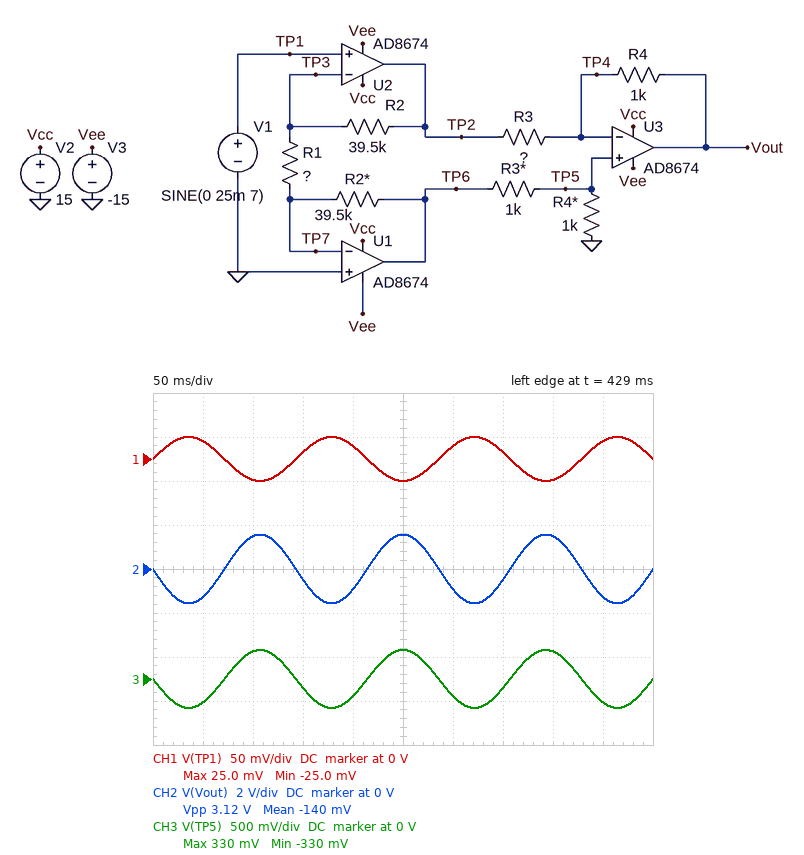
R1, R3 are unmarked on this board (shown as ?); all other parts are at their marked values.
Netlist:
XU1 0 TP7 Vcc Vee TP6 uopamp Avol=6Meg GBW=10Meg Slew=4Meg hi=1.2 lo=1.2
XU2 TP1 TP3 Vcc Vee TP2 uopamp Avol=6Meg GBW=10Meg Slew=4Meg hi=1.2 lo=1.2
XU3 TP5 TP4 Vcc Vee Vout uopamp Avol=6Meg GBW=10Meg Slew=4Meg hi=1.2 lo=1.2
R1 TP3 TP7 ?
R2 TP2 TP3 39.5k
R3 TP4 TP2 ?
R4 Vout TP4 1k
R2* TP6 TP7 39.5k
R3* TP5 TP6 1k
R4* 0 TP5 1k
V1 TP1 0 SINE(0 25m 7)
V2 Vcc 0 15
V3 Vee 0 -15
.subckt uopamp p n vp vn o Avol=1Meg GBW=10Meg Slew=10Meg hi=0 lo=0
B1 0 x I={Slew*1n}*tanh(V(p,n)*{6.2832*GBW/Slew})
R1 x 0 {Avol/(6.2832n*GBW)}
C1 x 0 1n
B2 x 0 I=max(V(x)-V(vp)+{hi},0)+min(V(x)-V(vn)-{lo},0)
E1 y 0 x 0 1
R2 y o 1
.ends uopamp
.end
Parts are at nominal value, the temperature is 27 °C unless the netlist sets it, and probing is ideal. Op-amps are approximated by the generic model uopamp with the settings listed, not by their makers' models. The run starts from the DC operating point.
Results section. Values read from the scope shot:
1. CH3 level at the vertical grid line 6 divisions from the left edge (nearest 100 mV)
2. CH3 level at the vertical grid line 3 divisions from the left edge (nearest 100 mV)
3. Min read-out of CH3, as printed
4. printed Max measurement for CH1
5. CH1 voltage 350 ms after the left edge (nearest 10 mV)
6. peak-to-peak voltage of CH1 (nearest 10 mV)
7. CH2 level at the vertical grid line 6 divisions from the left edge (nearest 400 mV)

-200 mV
-100 mV
-330 mV
25.0 mV
10 mV
50 mV
-800 mV
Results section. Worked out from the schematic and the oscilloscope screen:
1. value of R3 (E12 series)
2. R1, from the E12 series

820 Ω
1.5 kΩ
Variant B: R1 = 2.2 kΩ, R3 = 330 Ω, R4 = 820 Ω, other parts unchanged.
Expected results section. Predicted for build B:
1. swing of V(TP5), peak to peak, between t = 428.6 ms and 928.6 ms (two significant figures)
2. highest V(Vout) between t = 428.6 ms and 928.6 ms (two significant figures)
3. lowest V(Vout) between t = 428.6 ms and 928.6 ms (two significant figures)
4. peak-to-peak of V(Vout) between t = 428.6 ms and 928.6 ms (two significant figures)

450 mV
2.0 V
-2.0 V
3.9 V
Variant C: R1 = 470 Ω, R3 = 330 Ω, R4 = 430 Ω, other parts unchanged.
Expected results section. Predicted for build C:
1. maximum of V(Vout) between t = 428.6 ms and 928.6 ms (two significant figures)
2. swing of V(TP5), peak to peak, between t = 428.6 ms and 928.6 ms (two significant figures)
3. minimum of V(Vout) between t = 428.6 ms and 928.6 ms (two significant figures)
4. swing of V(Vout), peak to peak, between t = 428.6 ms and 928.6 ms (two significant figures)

5.2 V
2.1 V
-5.2 V
10 V
